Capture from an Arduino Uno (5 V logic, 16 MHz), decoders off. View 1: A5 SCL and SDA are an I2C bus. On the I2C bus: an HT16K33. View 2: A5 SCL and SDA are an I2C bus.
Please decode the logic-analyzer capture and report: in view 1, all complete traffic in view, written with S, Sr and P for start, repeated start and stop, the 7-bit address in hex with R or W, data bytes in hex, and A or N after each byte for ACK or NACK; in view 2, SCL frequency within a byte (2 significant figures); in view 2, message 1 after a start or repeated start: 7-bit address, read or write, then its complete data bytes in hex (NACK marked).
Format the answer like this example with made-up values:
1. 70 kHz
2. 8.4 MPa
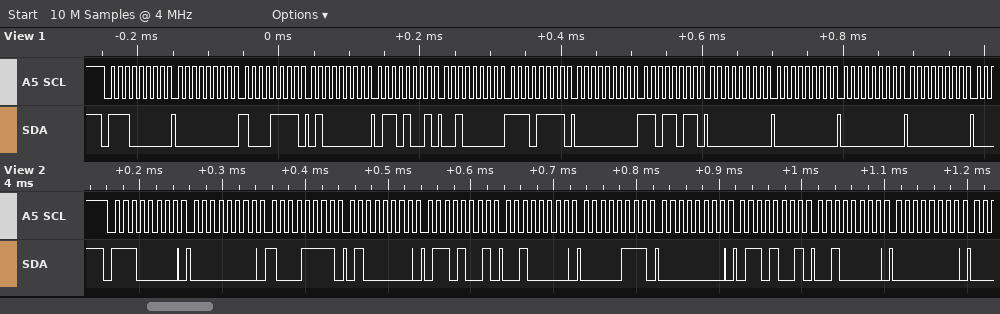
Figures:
1. S 70W A 00 A 8F A 40 A 69 A 20 A EF A 00 A DB A 00 A 00 A 00 A 00 A
2. 100 kHz
3. 0x70 write: 00 8F 40 69 20 07 00 69 20 00
